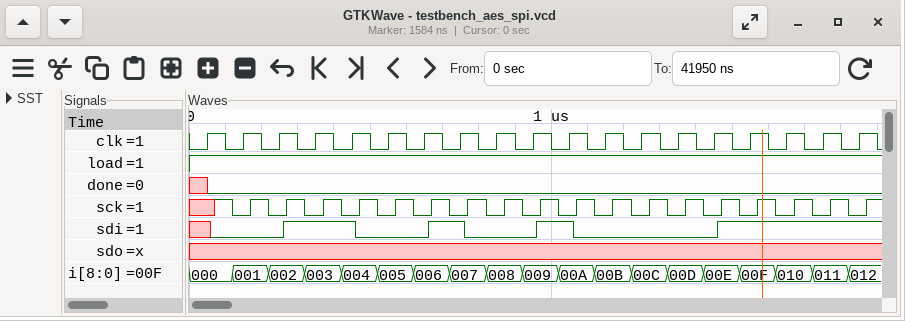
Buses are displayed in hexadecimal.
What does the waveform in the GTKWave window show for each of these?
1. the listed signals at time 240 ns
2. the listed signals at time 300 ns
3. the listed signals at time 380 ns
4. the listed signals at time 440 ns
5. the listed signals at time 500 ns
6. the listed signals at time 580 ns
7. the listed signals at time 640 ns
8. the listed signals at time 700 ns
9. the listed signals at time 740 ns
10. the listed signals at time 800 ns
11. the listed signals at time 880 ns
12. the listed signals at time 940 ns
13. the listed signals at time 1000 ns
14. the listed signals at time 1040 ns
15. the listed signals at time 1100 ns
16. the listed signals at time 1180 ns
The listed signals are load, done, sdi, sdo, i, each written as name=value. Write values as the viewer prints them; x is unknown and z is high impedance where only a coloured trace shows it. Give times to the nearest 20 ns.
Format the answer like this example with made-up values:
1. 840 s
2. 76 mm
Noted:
1. load=1, done=0, sdi=0, sdo=x, i=002
2. load=1, done=0, sdi=1, sdo=x, i=002
3. load=1, done=0, sdi=1, sdo=x, i=003
4. load=1, done=0, sdi=1, sdo=x, i=004
5. load=1, done=0, sdi=0, sdo=x, i=004
6. load=1, done=0, sdi=0, sdo=x, i=005
7. load=1, done=0, sdi=0, sdo=x, i=006
8. load=1, done=0, sdi=1, sdo=x, i=006
9. load=1, done=0, sdi=1, sdo=x, i=007
10. load=1, done=0, sdi=0, sdo=x, i=007
11. load=1, done=0, sdi=0, sdo=x, i=008
12. load=1, done=0, sdi=0, sdo=x, i=009
13. load=1, done=0, sdi=1, sdo=x, i=009
14. load=1, done=0, sdi=1, sdo=x, i=00A
15. load=1, done=0, sdi=0, sdo=x, i=00A
16. load=1, done=0, sdi=0, sdo=x, i=00B
